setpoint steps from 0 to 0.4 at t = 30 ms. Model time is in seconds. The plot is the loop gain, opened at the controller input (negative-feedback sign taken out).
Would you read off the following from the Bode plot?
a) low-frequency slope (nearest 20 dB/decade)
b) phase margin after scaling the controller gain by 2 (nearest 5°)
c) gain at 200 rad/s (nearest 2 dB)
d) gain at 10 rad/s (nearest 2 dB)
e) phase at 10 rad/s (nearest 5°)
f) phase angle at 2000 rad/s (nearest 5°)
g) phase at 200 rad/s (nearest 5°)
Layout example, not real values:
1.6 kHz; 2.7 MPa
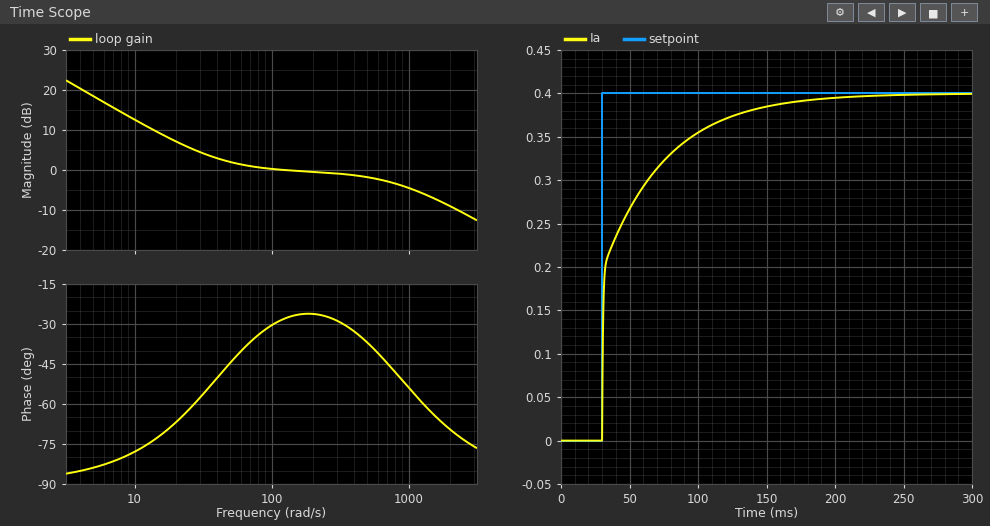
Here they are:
-20 dB/decade; 120°; 0 dB; 12 dB; -80°; -70°; -25°
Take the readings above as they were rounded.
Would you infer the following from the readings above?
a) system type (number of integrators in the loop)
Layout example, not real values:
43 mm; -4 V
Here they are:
1
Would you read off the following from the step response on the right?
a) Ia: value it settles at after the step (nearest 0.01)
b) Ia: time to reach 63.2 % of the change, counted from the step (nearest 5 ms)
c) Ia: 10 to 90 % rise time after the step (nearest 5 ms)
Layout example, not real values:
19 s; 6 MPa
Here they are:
0.40; 15 ms; 75 ms
